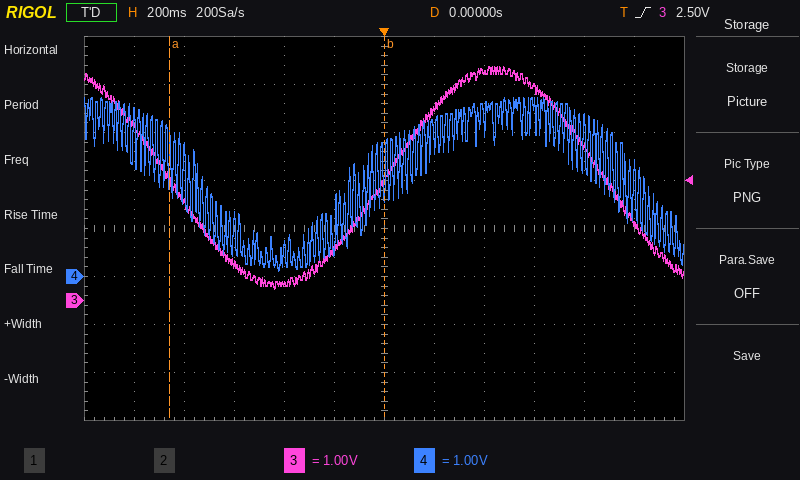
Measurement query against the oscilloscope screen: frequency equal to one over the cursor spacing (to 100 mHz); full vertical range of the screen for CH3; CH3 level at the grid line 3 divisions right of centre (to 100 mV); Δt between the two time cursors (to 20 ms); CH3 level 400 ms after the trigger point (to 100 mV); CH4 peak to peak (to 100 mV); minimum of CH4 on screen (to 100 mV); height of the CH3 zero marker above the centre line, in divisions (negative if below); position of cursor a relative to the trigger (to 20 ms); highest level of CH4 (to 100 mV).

1.2 Hz
8 V
4.4 V
860 ms
4.8 V
3.6 V
100 mV
-1.5 div
-860 ms
3.7 V
